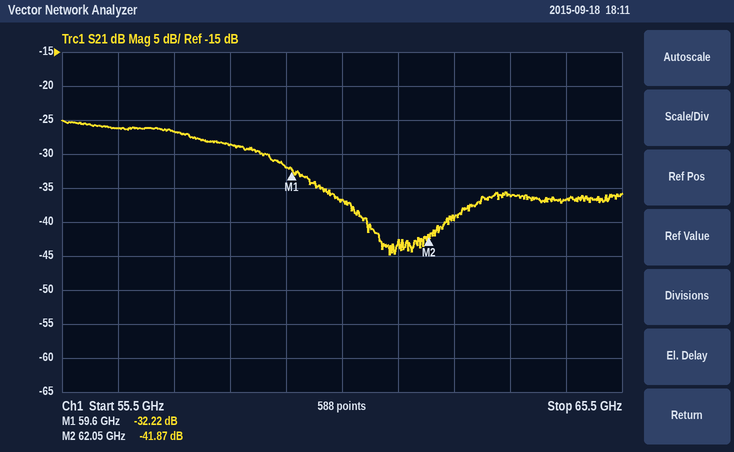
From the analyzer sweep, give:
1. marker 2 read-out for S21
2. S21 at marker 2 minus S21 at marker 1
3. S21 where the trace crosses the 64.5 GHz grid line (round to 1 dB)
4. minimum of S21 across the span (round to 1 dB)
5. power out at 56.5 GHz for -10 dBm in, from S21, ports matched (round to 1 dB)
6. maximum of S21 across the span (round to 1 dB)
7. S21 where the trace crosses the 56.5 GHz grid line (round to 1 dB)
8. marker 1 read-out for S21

-41.87 dB
-9.65 dB
-37 dB
-45 dB
-36 dBm
-25 dB
-26 dB
-32.22 dB
